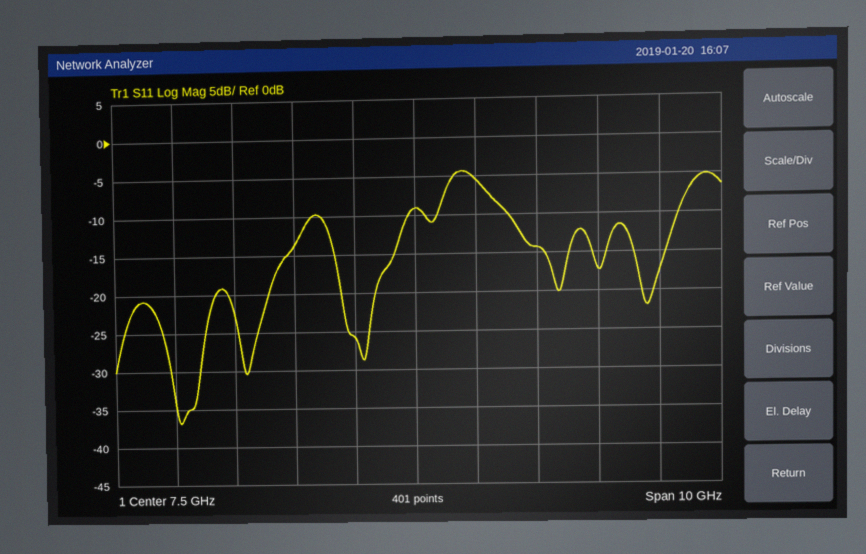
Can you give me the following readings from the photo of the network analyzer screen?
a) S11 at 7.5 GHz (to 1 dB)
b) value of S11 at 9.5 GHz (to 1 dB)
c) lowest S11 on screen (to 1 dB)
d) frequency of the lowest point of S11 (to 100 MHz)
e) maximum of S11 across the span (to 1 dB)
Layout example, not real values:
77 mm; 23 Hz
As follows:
-9 dB; -14 dB; -37 dB; 3.6 GHz; -4 dB
